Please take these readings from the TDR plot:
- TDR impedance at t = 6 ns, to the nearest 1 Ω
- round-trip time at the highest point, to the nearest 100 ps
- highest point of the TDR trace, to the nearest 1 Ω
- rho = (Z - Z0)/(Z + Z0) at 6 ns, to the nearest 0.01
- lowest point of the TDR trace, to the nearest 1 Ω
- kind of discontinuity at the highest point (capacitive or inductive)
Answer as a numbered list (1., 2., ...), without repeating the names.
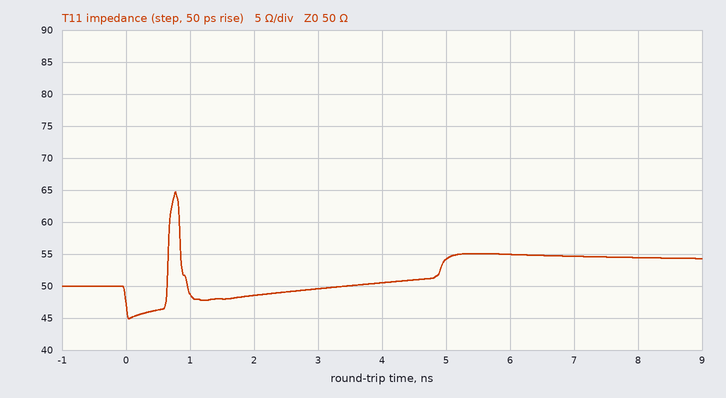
1. 55 Ω
2. 800 ps
3. 65 Ω
4. +0.05
5. 45 Ω
6. inductive
